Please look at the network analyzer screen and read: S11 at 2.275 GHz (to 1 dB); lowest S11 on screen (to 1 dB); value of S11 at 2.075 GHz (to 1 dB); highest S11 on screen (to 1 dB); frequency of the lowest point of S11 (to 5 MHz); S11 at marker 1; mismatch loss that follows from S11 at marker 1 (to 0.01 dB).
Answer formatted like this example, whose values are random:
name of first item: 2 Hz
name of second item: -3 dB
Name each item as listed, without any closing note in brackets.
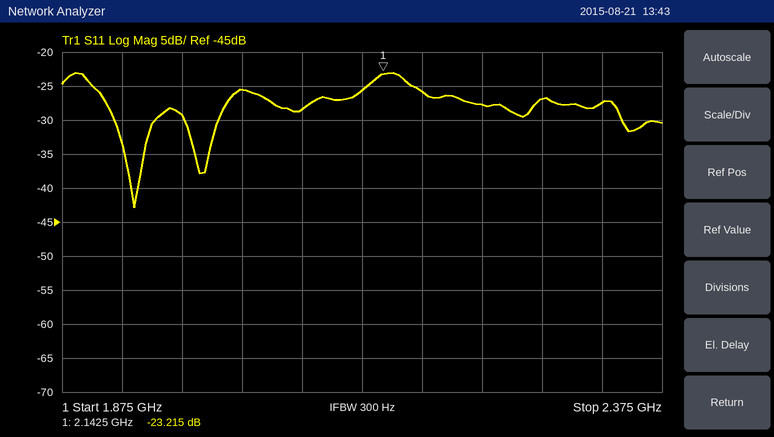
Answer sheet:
S11 at 2.275 GHz: -27 dB
lowest S11 on screen: -43 dB
value of S11 at 2.075 GHz: -28 dB
highest S11 on screen: -23 dB
frequency of the lowest point of S11: 1.935 GHz
S11 at marker 1: -23.215 dB
mismatch loss that follows from S11 at marker 1: 0.02 dB
